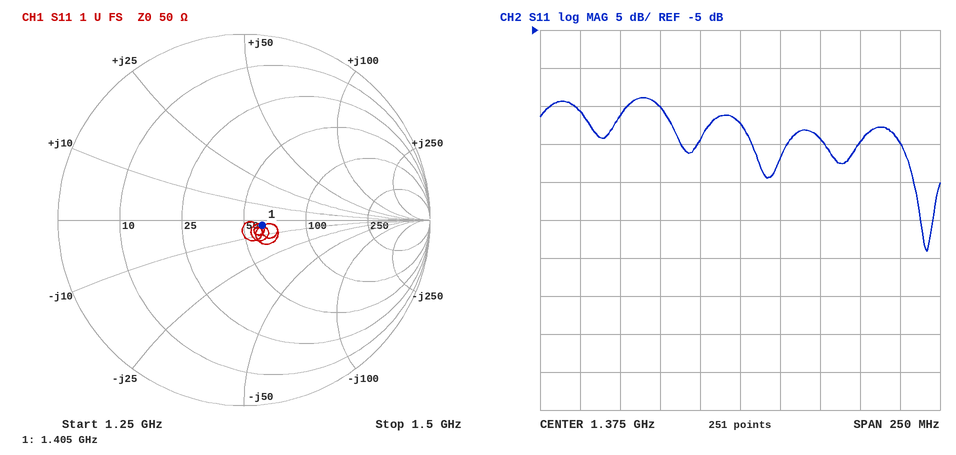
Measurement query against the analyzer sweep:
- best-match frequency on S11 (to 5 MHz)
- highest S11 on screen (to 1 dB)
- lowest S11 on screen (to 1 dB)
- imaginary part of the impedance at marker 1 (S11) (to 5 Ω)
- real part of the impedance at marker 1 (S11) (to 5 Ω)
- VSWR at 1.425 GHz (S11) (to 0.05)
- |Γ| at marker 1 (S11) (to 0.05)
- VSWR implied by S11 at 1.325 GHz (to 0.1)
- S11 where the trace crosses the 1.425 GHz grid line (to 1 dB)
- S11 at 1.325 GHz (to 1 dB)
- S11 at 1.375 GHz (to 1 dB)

1.490 GHz
-14 dB
-34 dB
-5 Ω
60 Ω
1.25
0.10
1.4
-19 dB
-15 dB
-17 dB
